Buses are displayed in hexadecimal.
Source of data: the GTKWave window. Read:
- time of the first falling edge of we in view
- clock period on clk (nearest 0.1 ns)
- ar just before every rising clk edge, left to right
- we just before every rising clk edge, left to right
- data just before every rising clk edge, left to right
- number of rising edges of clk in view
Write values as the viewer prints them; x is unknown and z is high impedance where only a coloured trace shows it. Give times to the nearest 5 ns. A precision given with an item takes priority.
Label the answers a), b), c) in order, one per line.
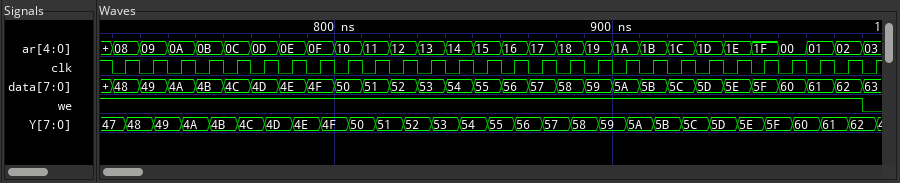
a) 990 ns
b) 10 ns
c) 08, 09, 0A, 0B, 0C, 0D, 0E, 0F, 10, 11, 12, 13, 14, 15, 16, 17, 18, 19, 1A, 1B, 1C, 1D, 1E, 1F, 00, 01, 02, 03
d) 1 1 1 1 1 1 1 1 1 1 1 1 1 1 1 1 1 1 1 1 1 1 1 1 1 1 1 0
e) 48, 49, 4A, 4B, 4C, 4D, 4E, 4F, 50, 51, 52, 53, 54, 55, 56, 57, 58, 59, 5A, 5B, 5C, 5D, 5E, 5F, 60, 61, 62, 63
f) 28
